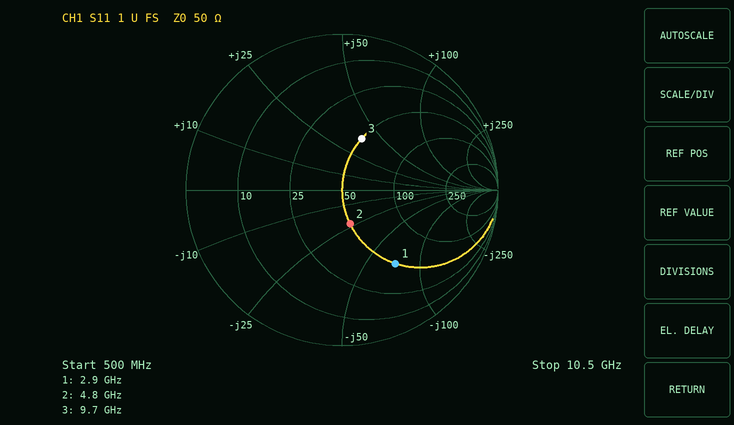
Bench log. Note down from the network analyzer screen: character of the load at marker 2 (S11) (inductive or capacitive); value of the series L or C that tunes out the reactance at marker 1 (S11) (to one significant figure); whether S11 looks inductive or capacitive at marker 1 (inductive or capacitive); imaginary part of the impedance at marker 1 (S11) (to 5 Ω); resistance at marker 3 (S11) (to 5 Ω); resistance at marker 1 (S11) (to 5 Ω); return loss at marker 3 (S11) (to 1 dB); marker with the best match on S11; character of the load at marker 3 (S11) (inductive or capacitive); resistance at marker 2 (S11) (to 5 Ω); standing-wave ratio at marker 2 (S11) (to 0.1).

capacitive
4 nH
capacitive
-70 Ω
50 Ω
50 Ω
9 dB
marker 2
inductive
50 Ω
1.6
